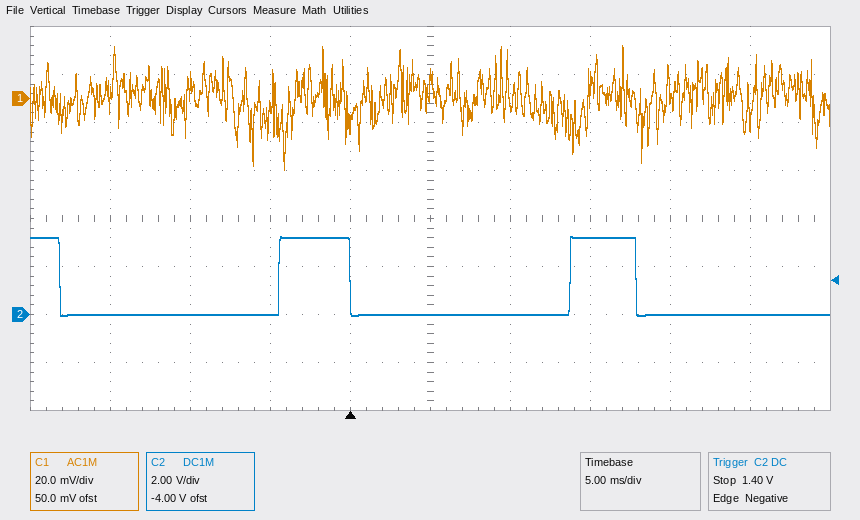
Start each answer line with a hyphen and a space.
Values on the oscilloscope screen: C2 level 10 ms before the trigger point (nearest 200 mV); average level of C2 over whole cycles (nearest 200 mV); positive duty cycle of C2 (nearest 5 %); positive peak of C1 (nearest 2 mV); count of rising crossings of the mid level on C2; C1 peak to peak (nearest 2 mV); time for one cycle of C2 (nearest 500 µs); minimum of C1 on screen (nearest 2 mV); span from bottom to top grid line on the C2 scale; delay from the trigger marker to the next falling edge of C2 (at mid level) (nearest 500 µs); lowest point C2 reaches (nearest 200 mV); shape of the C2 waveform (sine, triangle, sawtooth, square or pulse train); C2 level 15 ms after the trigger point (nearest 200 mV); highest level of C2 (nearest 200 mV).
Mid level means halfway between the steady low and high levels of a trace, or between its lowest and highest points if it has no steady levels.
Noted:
- 0.0 V
- 800 mV
- 25 %
- 22 mV
- 2
- 52 mV
- 18.0 ms
- -30 mV
- 16 V
- 18.0 ms
- 0.0 V
- pulse train
- 3.2 V
- 3.2 V
